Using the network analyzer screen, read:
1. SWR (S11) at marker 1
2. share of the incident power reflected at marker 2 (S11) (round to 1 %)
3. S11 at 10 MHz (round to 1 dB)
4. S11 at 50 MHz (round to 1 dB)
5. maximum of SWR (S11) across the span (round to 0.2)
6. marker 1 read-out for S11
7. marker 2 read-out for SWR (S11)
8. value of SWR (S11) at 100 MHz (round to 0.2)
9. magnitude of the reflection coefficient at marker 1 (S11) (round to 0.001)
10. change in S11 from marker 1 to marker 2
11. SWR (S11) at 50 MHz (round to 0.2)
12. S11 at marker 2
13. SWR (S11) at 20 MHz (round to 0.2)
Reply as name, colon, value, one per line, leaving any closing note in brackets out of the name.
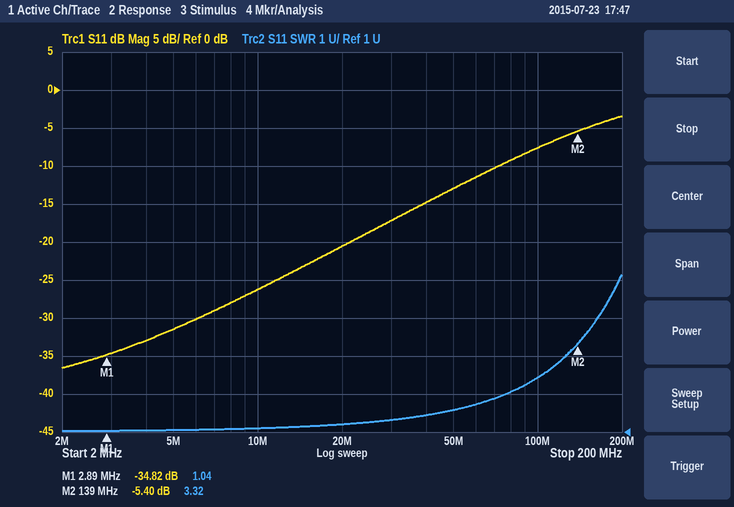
SWR (S11) at marker 1: 1.04
share of the incident power reflected at marker 2 (S11): 29 %
S11 at 10 MHz: -26 dB
S11 at 50 MHz: -13 dB
maximum of SWR (S11) across the span: 5.2
marker 1 read-out for S11: -34.82 dB
marker 2 read-out for SWR: 3.32
value of SWR (S11) at 100 MHz: 2.4
magnitude of the reflection coefficient at marker 1 (S11): 0.018
change in S11 from marker 1 to marker 2: 29.42 dB
SWR (S11) at 50 MHz: 1.6
S11 at marker 2: -5.40 dB
SWR (S11) at 20 MHz: 1.2
